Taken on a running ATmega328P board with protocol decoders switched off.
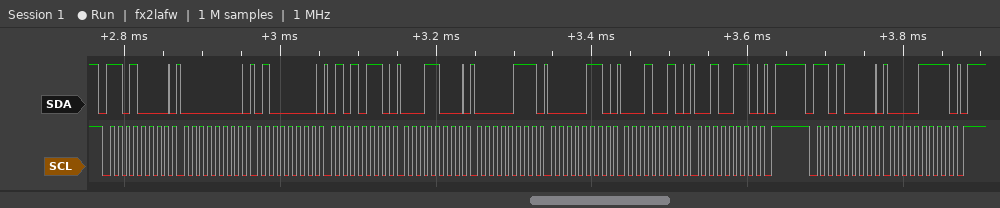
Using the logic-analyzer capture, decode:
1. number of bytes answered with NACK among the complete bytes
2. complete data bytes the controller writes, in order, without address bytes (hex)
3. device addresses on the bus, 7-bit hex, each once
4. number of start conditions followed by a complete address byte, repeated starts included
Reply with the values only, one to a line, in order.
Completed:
0
00 40 56 18 07 06 12 26 0F
0x68
2
